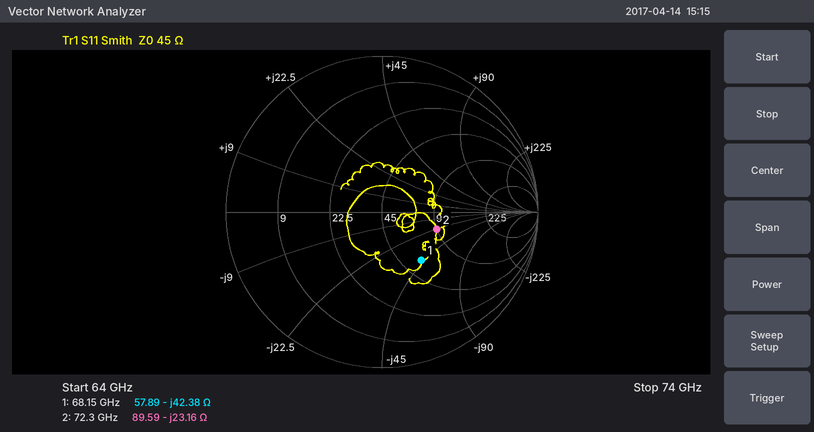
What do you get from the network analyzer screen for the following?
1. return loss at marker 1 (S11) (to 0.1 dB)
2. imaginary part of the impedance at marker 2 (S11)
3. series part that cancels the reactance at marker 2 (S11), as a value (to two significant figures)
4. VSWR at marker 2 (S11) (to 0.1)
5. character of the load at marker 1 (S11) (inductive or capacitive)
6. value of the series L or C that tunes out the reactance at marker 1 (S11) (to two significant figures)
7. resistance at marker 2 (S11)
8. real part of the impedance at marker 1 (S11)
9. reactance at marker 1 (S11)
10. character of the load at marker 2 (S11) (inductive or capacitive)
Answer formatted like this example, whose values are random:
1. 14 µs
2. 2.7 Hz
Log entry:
1. 8.0 dB
2. -23.16 Ω
3. 51 pH
4. 2.2
5. capacitive
6. 99 pH
7. 89.59 Ω
8. 57.89 Ω
9. -42.38 Ω
10. capacitive
